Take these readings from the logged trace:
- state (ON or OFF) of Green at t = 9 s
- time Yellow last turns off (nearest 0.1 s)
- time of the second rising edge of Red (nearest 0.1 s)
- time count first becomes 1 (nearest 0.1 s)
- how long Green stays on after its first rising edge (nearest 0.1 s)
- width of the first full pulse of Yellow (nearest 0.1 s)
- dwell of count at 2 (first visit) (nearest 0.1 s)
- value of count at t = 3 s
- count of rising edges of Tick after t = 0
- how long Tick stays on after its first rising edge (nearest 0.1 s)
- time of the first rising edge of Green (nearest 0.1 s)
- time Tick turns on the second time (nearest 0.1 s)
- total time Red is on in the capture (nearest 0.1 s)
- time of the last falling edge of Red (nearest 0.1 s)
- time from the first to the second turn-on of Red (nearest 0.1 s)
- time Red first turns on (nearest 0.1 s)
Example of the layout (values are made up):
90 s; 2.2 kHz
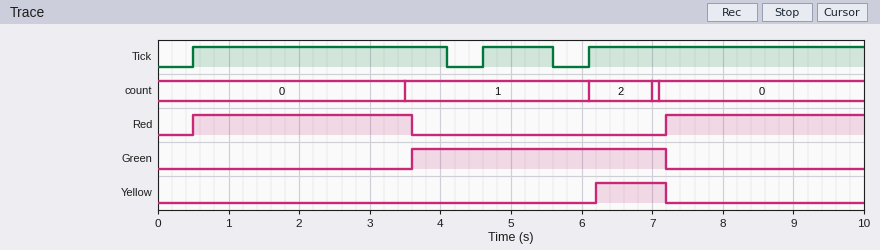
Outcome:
OFF; 7.2 s; 7.2 s; 3.5 s; 3.6 s; 1.0 s; 0.9 s; 0; 3; 3.6 s; 3.6 s; 4.6 s; 5.9 s; 3.6 s; 6.7 s; 0.5 s
